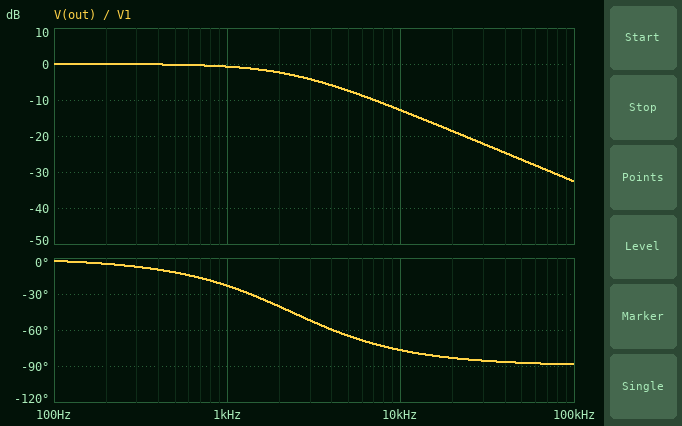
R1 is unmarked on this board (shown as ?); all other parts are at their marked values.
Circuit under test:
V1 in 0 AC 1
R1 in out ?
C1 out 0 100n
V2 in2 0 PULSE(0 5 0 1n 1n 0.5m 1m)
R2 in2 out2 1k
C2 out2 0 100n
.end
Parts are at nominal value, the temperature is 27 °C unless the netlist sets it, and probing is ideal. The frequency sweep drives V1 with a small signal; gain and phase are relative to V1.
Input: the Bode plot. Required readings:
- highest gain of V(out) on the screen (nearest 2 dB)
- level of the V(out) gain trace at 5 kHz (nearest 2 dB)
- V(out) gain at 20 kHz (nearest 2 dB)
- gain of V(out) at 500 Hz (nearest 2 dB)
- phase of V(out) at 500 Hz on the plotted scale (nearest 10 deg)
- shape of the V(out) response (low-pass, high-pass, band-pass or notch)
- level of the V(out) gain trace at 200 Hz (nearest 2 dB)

0 dB
-8 dB
-18 dB
0 dB
-10 deg
low-pass
0 dB
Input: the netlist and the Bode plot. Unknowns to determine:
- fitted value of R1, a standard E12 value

680 Ω
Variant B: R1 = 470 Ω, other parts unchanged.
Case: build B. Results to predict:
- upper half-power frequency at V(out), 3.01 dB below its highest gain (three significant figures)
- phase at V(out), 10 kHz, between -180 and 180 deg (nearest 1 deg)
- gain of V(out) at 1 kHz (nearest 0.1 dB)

3.39 kHz
-71 deg
-0.4 dB
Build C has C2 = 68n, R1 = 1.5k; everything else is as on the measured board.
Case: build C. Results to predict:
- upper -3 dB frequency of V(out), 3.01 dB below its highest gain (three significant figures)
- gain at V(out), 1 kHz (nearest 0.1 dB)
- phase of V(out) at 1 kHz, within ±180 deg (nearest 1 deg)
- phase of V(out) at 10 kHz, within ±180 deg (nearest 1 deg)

1.06 kHz
-2.8 dB
-43 deg
-84 deg
